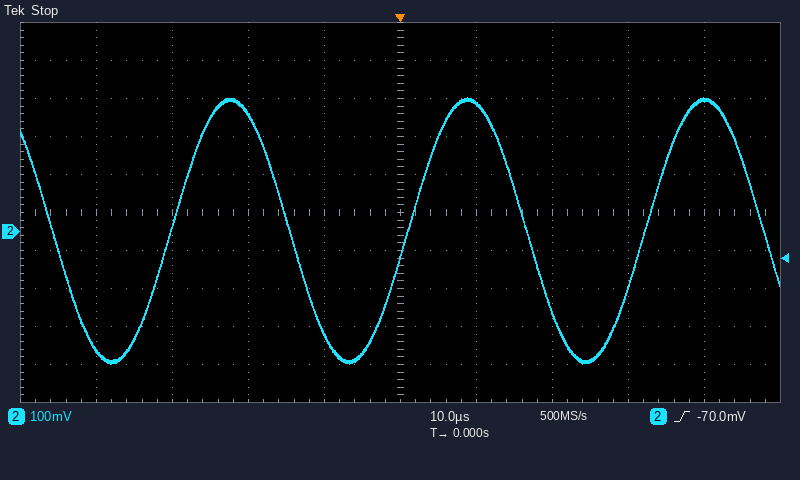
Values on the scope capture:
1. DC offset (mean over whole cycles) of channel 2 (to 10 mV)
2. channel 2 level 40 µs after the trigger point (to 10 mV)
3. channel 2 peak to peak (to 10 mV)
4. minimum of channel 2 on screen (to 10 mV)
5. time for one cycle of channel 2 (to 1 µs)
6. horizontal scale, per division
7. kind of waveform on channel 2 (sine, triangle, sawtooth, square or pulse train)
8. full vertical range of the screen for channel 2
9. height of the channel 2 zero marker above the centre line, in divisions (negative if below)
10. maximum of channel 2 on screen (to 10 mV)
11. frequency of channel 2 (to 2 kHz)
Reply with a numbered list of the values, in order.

1. 0 mV
2. 350 mV
3. 700 mV
4. -350 mV
5. 31 µs
6. 10 µs
7. sine
8. 1 V
9. -0.5 div
10. 350 mV
11. 32 kHz
